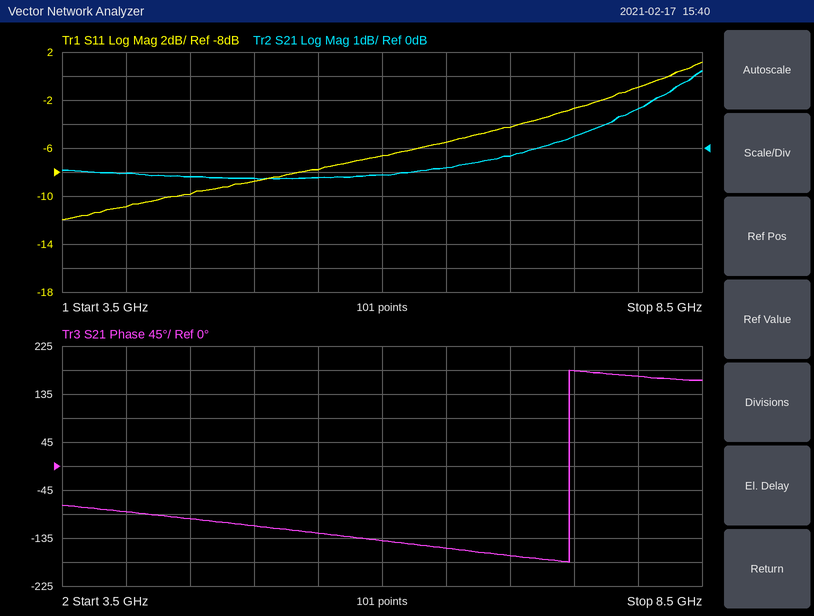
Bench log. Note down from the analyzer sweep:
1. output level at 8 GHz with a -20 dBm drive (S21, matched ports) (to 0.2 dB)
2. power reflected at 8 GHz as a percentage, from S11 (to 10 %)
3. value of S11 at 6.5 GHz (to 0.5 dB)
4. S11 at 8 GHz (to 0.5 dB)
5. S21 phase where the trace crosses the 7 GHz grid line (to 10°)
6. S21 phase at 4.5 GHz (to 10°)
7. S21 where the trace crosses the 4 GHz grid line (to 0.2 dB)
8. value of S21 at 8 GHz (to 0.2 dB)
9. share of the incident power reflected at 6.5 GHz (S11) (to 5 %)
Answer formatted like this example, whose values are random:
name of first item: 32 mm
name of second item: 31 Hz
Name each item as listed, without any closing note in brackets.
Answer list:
output level at 8 GHz with a -20 dBm drive (S21, matched ports): -18.4 dBm
power reflected at 8 GHz as a percentage, from S11: 80 %
value of S11 at 6.5 GHz: -5.5 dB
S11 at 8 GHz: -1.0 dB
S21 phase where the trace crosses the 7 GHz grid line: -170°
S21 phase at 4.5 GHz: -100°
S21 where the trace crosses the 4 GHz grid line: -1.0 dB
value of S21 at 8 GHz: 1.6 dB
share of the incident power reflected at 6.5 GHz (S11): 30 %
